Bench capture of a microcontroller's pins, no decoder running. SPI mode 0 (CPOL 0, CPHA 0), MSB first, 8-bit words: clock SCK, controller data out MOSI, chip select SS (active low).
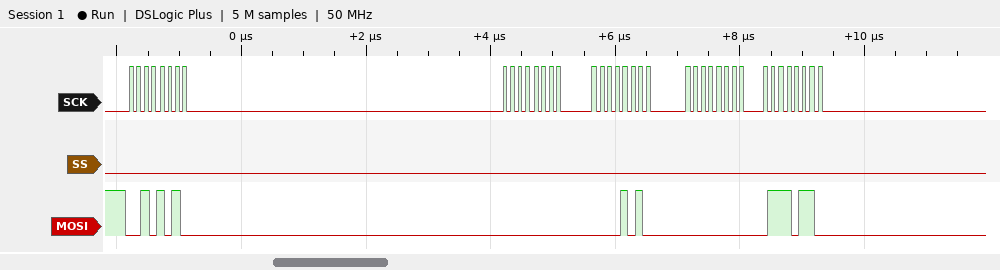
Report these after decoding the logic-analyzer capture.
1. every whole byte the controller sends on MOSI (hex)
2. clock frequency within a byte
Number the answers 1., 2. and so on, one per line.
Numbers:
1. 0x2A 0x00 0x0A 0x00 0x76
2. 8 MHz
